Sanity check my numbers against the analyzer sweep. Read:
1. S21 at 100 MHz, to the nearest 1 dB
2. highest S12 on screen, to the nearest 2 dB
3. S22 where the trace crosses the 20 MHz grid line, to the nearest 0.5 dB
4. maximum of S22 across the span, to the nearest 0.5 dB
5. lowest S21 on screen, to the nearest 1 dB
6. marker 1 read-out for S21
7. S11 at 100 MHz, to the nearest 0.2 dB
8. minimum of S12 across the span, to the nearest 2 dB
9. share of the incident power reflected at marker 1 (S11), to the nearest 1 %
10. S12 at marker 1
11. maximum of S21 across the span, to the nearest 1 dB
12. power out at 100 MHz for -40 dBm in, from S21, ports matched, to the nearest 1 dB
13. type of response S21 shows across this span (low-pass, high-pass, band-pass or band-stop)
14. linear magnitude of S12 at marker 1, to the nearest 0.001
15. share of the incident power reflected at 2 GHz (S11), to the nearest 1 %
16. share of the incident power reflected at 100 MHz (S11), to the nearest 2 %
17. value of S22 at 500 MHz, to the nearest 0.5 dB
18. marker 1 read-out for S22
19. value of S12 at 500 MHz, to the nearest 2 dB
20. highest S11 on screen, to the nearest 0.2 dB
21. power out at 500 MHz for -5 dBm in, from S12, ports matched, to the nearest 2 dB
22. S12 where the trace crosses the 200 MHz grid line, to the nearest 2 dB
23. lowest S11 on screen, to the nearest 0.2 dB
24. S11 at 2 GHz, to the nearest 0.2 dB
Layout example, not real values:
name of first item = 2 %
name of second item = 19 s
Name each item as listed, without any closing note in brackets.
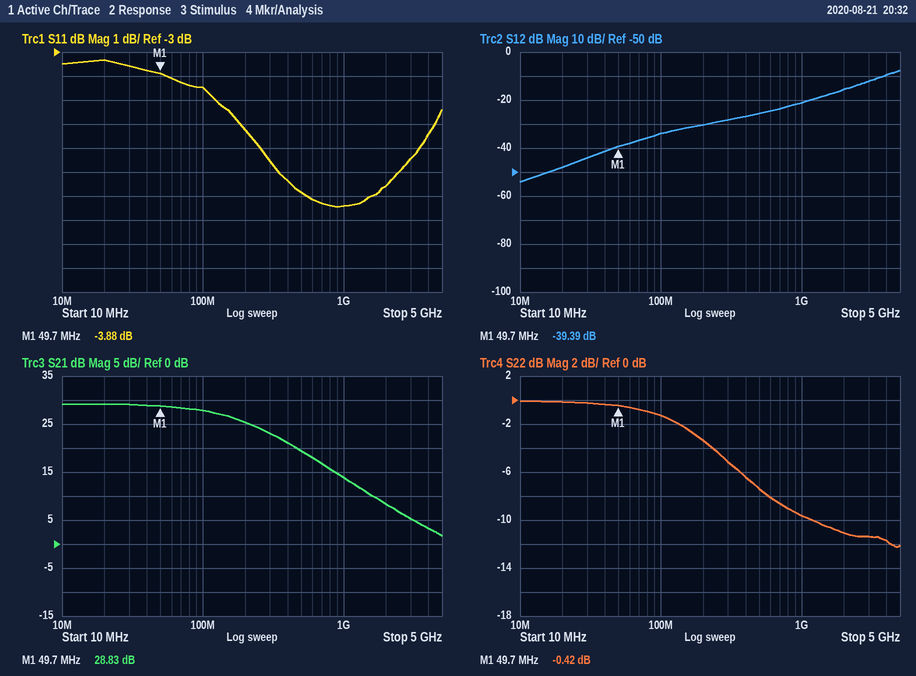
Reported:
S21 at 100 MHz, to the nearest 1 dB = 28 dB
highest S12 on screen, to the nearest 2 dB = -8 dB
S22 where the trace crosses the 20 MHz grid line, to the nearest 0.5 dB = 0.0 dB
maximum of S22 across the span, to the nearest 0.5 dB = 0.0 dB
lowest S21 on screen, to the nearest 1 dB = 2 dB
marker 1 read-out for S21 = 28.83 dB
S11 at 100 MHz, to the nearest 0.2 dB = -4.4 dB
minimum of S12 across the span, to the nearest 2 dB = -54 dB
share of the incident power reflected at marker 1 (S11), to the nearest 1 % = 41 %
S12 at marker 1 = -39.39 dB
maximum of S21 across the span, to the nearest 1 dB = 29 dB
power out at 100 MHz for -40 dBm in, from S21, ports matched, to the nearest 1 dB = -12 dBm
type of response S21 shows across this span = low-pass
linear magnitude of S12 at marker 1, to the nearest 0.001 = 0.011
share of the incident power reflected at 2 GHz (S11), to the nearest 1 % = 14 %
share of the incident power reflected at 100 MHz (S11), to the nearest 2 % = 36 %
value of S22 at 500 MHz, to the nearest 0.5 dB = -7.5 dB
marker 1 read-out for S22 = -0.42 dB
value of S12 at 500 MHz, to the nearest 2 dB = -26 dB
highest S11 on screen, to the nearest 0.2 dB = -3.4 dB
power out at 500 MHz for -5 dBm in, from S12, ports matched, to the nearest 2 dB = -30 dBm
S12 where the trace crosses the 200 MHz grid line, to the nearest 2 dB = -30 dB
lowest S11 on screen, to the nearest 0.2 dB = -9.4 dB
S11 at 2 GHz, to the nearest 0.2 dB = -8.6 dB
